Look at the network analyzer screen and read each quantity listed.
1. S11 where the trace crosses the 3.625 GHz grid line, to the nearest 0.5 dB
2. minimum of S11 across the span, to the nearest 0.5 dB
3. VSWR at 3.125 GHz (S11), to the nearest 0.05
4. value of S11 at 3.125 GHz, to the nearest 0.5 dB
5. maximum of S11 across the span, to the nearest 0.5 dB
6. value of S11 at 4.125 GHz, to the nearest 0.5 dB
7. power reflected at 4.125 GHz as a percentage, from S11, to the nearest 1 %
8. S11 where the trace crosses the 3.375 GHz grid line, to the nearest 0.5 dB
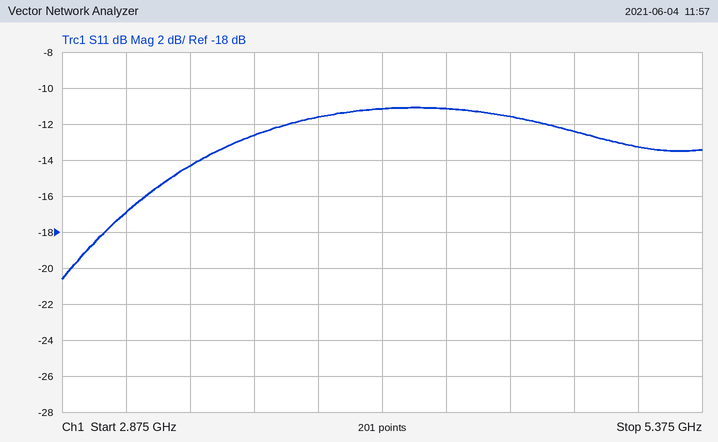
-12.5 dB
-20.5 dB
1.35
-17.0 dB
-11.0 dB
-11.0 dB
8 %
-14.5 dB
